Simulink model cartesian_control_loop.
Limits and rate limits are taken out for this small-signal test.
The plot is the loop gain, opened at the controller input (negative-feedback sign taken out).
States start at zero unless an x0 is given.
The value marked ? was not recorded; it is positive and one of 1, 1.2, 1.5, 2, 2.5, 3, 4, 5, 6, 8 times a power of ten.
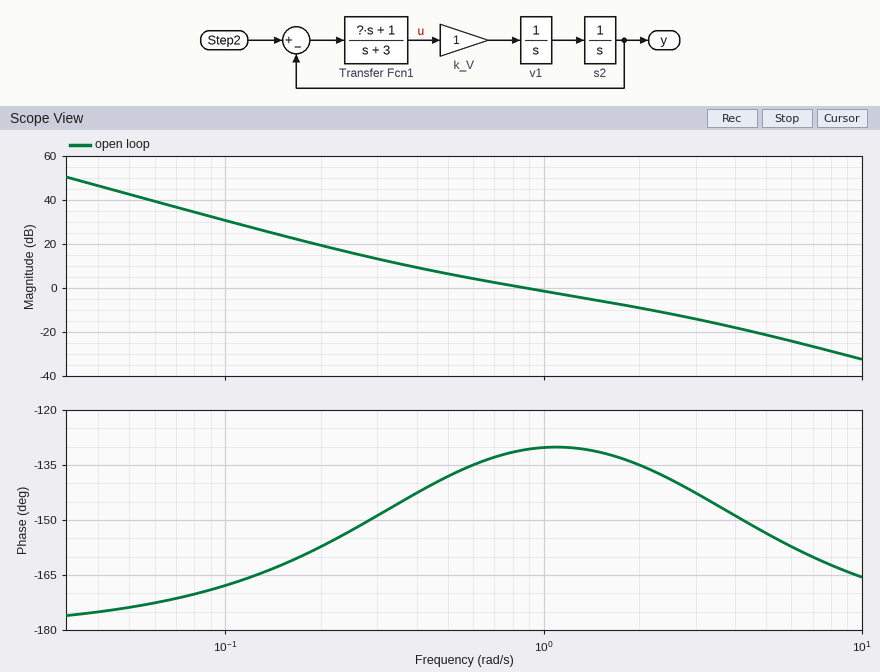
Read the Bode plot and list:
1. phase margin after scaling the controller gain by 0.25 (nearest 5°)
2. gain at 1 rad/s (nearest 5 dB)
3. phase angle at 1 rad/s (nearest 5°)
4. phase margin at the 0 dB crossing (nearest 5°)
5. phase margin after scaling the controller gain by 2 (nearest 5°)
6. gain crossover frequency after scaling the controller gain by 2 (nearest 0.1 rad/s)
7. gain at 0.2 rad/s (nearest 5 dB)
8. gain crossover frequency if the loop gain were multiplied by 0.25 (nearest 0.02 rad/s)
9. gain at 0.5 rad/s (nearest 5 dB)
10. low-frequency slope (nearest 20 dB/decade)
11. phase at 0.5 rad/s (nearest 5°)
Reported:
35°
0 dB
-130°
50°
50°
1.5 rad/s
20 dB
0.32 rad/s
5 dB
-40 dB/decade
-140°
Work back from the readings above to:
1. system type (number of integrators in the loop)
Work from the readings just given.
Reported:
2
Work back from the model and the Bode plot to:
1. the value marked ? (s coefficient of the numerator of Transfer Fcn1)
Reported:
2.5
